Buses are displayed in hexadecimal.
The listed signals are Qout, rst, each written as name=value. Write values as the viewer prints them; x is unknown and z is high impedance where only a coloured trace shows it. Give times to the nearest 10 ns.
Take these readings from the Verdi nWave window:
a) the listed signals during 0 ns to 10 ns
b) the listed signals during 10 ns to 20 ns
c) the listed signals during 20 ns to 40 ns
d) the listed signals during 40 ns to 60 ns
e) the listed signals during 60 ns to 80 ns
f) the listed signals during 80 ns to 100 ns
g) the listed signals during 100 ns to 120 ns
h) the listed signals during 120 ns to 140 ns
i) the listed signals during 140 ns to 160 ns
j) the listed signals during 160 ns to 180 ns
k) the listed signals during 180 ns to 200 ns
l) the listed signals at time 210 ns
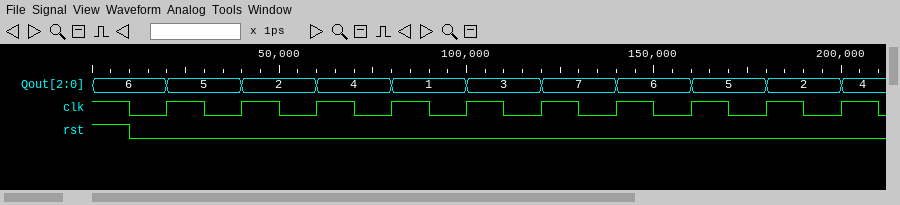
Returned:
Qout=6, rst=1
Qout=6, rst=0
Qout=5, rst=0
Qout=2, rst=0
Qout=4, rst=0
Qout=1, rst=0
Qout=3, rst=0
Qout=7, rst=0
Qout=6, rst=0
Qout=5, rst=0
Qout=2, rst=0
Qout=4, rst=0
